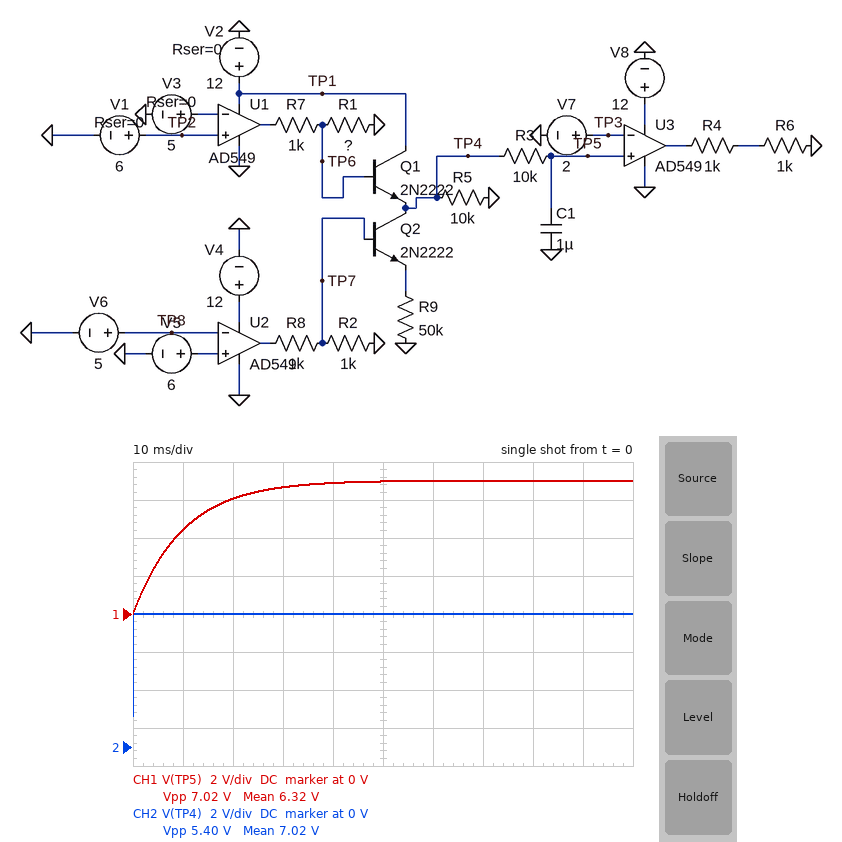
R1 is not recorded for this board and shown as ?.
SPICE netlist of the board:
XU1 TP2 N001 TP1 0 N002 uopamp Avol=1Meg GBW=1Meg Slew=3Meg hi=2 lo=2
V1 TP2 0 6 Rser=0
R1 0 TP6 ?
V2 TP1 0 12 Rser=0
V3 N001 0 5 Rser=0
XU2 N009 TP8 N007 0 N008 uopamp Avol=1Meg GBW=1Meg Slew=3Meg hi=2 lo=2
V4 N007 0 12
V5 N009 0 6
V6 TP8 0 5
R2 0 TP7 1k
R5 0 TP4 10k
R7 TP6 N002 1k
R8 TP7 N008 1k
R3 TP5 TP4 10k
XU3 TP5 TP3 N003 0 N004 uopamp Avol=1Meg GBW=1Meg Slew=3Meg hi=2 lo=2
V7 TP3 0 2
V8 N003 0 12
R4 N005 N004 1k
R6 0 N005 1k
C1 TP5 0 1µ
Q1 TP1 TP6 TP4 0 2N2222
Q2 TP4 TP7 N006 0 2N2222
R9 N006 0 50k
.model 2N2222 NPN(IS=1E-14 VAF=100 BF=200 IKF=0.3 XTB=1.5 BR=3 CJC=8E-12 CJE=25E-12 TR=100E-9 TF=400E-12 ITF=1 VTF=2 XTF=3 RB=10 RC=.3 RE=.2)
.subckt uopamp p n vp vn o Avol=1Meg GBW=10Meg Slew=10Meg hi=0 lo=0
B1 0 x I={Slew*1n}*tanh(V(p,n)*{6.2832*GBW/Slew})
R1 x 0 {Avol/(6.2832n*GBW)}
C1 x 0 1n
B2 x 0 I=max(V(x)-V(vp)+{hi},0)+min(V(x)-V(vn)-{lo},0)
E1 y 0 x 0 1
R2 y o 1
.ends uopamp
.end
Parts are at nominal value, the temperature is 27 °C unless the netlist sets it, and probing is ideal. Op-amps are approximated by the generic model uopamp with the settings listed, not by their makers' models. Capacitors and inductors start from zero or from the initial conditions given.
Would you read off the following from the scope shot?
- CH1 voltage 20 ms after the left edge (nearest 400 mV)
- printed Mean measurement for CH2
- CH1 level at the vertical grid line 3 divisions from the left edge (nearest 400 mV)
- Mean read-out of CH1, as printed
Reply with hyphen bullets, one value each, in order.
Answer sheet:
- 6.0 V
- 7.02 V
- 6.8 V
- 6.32 V
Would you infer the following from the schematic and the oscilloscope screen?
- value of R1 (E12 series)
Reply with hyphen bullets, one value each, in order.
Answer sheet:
- 3.3 kΩ
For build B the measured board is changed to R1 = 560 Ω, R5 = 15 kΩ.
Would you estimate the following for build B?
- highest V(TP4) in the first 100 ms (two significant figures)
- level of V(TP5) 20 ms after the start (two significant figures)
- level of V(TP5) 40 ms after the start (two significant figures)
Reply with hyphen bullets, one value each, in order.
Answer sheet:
- 4.2 V
- 3.5 V
- 4.1 V
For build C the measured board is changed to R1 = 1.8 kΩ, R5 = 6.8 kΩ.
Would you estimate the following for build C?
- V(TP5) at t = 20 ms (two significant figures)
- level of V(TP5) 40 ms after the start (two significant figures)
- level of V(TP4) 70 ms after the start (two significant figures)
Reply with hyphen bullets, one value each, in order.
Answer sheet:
- 5.0 V
- 5.7 V
- 5.8 V
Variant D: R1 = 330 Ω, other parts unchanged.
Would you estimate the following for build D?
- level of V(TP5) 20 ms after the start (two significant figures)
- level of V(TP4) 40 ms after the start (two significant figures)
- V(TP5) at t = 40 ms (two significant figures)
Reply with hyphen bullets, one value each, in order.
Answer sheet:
- 3.5 V
- 4.1 V
- 4.0 V
